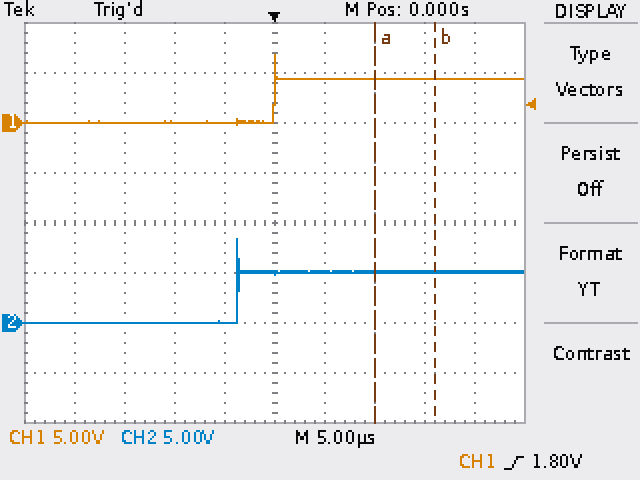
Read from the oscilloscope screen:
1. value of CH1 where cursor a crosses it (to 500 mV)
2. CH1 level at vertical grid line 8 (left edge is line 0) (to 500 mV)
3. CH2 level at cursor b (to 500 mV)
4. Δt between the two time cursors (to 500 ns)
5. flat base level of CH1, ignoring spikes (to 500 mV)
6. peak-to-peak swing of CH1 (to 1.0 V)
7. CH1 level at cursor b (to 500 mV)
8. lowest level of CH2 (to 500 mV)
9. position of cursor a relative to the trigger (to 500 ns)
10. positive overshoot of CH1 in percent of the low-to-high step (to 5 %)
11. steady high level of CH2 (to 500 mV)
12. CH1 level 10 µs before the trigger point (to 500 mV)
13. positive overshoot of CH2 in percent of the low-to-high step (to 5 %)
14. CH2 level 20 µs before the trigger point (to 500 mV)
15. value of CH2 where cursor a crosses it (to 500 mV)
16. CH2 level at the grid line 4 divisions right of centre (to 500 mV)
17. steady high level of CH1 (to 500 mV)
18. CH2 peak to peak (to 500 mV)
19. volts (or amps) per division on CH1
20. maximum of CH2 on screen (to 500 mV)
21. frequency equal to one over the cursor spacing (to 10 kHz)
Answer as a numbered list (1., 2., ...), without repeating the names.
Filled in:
1. 4.5 V
2. 4.5 V
3. 5.0 V
4. 6.0 µs
5. 0.0 V
6. 7.0 V
7. 4.5 V
8. 0.0 V
9. +10.0 µs
10. 55 %
11. 5.0 V
12. 0.0 V
13. 65 %
14. 0.0 V
15. 5.0 V
16. 5.0 V
17. 4.5 V
18. 8.5 V
19. 5 V
20. 8.5 V
21. 170 kHz
